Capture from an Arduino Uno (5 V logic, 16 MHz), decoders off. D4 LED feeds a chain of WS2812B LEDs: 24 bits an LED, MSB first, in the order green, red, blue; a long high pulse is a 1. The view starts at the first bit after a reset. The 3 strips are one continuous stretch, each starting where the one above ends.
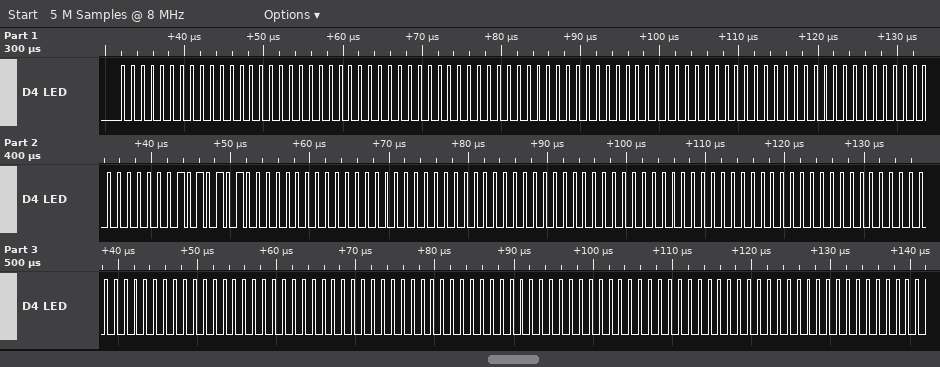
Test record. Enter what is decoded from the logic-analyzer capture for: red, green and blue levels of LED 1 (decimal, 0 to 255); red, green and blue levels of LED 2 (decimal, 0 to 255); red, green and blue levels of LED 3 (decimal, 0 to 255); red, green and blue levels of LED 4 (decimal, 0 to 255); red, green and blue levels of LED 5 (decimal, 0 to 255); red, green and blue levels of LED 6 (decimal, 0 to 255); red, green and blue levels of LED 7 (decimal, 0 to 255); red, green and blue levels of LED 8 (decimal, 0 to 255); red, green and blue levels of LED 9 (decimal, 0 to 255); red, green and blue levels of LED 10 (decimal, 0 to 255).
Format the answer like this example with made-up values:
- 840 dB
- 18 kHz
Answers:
- 0, 0, 0
- 0, 0, 0
- 0, 0, 0
- 0, 0, 85
- 0, 0, 0
- 0, 0, 0
- 0, 0, 0
- 0, 0, 0
- 0, 0, 0
- 0, 0, 0
